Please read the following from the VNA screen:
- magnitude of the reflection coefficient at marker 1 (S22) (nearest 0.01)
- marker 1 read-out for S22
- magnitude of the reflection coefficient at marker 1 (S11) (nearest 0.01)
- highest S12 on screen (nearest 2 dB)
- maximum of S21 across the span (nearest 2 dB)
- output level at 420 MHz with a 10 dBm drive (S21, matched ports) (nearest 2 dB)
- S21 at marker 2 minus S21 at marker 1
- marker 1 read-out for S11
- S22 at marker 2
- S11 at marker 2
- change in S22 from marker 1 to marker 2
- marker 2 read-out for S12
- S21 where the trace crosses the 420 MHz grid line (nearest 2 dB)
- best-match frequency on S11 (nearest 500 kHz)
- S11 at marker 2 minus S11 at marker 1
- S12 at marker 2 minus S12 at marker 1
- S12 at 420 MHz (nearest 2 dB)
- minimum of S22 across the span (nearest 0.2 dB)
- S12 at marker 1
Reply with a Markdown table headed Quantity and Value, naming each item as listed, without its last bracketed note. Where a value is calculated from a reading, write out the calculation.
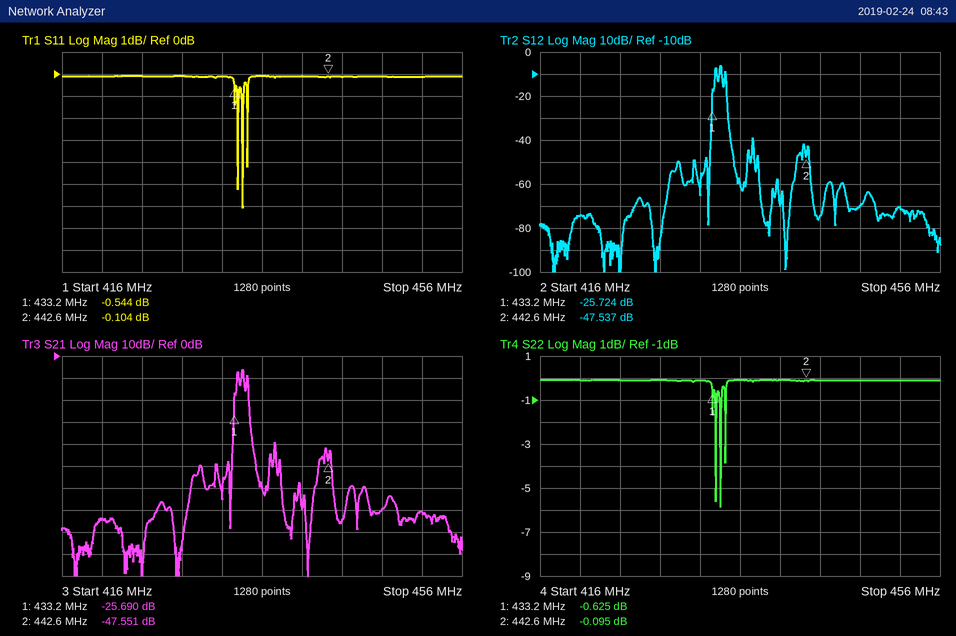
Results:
| Quantity | Value |
|---|---|
| magnitude of the reflection coefficient at marker 1 (S22) | 10^(-0.625/20) ≈ 0.93 |
| marker 1 read-out for S22 | -0.625 dB |
| magnitude of the reflection coefficient at marker 1 (S11) | 10^(-0.544/20) ≈ 0.94 |
| highest S12 on screen | -6 dB |
| maximum of S21 across the span | -6 dB |
| output level at 420 MHz with a 10 dBm drive (S21, matched ports) | 10 dBm + (-74 dB) = -64 dBm |
| S21 at marker 2 minus S21 at marker 1 | -47.551 − (-25.69) = -21.861 dB |
| marker 1 read-out for S11 | -0.544 dB |
| S22 at marker 2 | -0.095 dB |
| S11 at marker 2 | -0.104 dB |
| change in S22 from marker 1 to marker 2 | -0.095 − (-0.625) = 0.530 dB |
| marker 2 read-out for S12 | -47.537 dB |
| S21 where the trace crosses the 420 MHz grid line | -74 dB |
| best-match frequency on S11 | 434.0 MHz |
| S11 at marker 2 minus S11 at marker 1 | -0.104 − (-0.544) = 0.440 dB |
| S12 at marker 2 minus S12 at marker 1 | -47.537 − (-25.724) = -21.813 dB |
| S12 at 420 MHz | -74 dB |
| minimum of S22 across the span | -5.8 dB |
| S12 at marker 1 | -25.724 dB |
